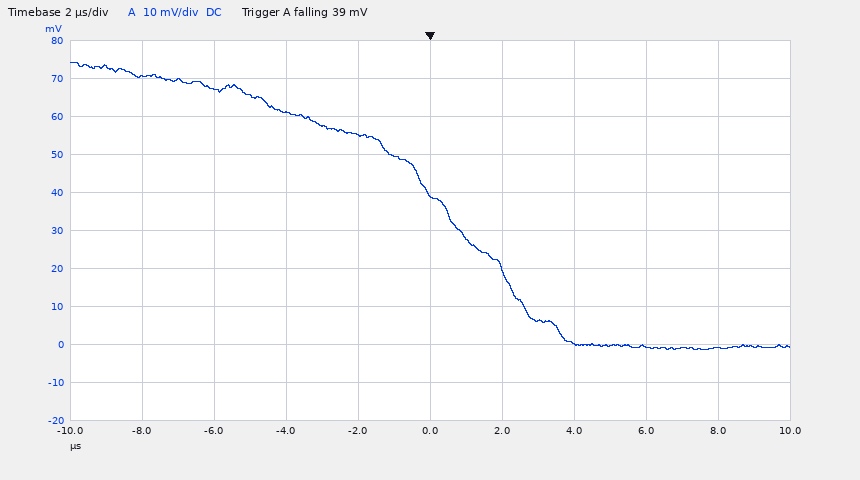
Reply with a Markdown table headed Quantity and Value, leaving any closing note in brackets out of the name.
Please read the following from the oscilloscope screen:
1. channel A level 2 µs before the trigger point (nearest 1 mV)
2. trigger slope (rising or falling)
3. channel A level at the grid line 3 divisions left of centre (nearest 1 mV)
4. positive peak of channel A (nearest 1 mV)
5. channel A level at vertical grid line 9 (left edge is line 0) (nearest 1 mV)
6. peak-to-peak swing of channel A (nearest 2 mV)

| Quantity | Value |
|---|---|
| channel A level 2 µs before the trigger point | 55 mV |
| trigger slope | falling |
| channel A level at the grid line 3 divisions left of centre | 67 mV |
| positive peak of channel A | 74 mV |
| channel A level at vertical grid line 9 (left edge is line 0) | -1 mV |
| peak-to-peak swing of channel A | 76 mV |
